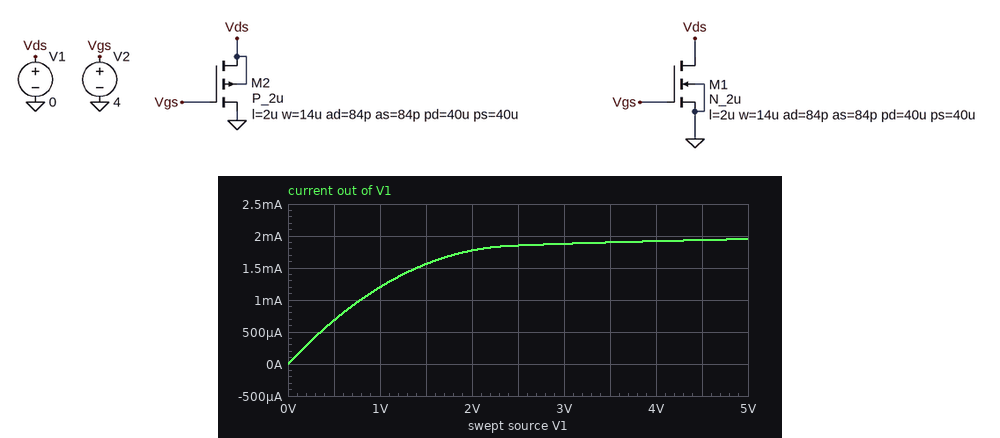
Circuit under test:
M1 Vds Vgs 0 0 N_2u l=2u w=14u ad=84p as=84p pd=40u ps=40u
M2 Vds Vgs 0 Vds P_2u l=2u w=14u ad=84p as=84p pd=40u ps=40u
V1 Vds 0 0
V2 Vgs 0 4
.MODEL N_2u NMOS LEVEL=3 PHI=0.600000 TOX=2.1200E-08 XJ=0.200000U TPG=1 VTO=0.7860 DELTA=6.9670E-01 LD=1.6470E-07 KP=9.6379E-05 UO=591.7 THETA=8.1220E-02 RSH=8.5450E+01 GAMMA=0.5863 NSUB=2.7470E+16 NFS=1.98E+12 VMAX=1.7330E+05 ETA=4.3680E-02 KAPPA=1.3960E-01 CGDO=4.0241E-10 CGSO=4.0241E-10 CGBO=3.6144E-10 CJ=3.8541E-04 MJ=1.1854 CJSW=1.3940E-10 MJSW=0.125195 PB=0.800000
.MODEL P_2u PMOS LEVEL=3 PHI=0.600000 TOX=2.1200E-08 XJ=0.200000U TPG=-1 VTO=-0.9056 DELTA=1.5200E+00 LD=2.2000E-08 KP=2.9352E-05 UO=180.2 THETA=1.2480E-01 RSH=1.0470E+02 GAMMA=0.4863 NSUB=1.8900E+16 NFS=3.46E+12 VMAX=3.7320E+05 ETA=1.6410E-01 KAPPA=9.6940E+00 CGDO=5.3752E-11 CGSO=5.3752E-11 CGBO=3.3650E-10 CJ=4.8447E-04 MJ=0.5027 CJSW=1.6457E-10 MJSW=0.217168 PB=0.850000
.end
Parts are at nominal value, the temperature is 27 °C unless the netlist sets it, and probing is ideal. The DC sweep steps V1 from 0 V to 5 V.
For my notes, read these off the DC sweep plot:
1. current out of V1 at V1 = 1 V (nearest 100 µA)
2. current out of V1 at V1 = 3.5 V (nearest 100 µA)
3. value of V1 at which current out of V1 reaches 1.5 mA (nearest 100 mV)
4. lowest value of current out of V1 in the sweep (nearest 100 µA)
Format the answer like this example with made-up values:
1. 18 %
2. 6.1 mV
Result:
1. 1.2 mA
2. 1.9 mA
3. 1.4 V
4. 0 A
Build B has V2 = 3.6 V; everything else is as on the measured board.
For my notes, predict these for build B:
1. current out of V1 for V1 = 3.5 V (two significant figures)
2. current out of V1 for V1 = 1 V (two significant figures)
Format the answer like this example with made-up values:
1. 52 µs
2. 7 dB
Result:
1. 1.6 mA
2. 1.1 mA
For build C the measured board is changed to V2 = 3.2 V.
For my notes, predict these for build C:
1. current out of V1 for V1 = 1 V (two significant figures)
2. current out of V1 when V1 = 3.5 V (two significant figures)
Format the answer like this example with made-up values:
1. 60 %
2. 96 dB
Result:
1. 920 µA
2. 1.2 mA
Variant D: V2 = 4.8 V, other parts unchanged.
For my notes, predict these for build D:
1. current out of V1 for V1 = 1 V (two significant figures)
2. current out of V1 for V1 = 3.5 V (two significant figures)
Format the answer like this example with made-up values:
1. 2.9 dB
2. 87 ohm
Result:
1. 1.4 mA
2. 2.6 mA
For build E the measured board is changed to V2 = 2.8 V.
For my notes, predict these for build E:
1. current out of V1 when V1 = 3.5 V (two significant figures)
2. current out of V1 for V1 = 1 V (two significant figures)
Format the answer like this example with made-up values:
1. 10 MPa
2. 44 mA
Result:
1. 930 µA
2. 760 µA
